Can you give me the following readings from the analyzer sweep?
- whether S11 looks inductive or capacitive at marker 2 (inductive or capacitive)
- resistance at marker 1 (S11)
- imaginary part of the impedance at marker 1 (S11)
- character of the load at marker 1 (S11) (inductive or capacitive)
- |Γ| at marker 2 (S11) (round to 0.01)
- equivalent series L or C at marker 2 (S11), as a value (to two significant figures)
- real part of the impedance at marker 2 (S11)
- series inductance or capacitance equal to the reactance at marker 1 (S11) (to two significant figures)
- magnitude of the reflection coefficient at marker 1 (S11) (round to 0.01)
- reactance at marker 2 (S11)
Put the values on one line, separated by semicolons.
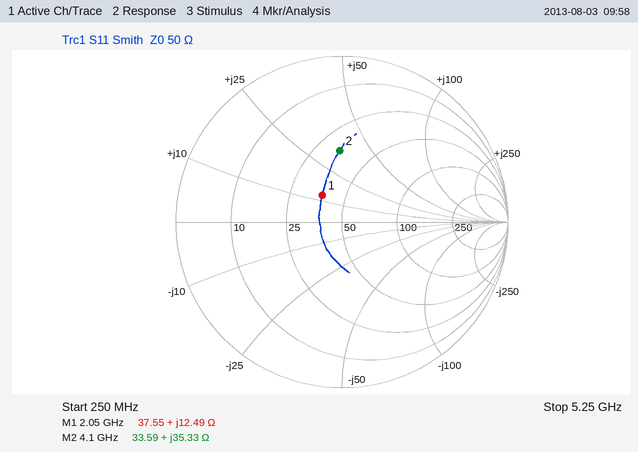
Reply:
inductive; 37.55 Ω; +12.49 Ω; inductive; 0.43; 1.4 nH; 33.59 Ω; 970 pH; 0.20; +35.33 Ω
